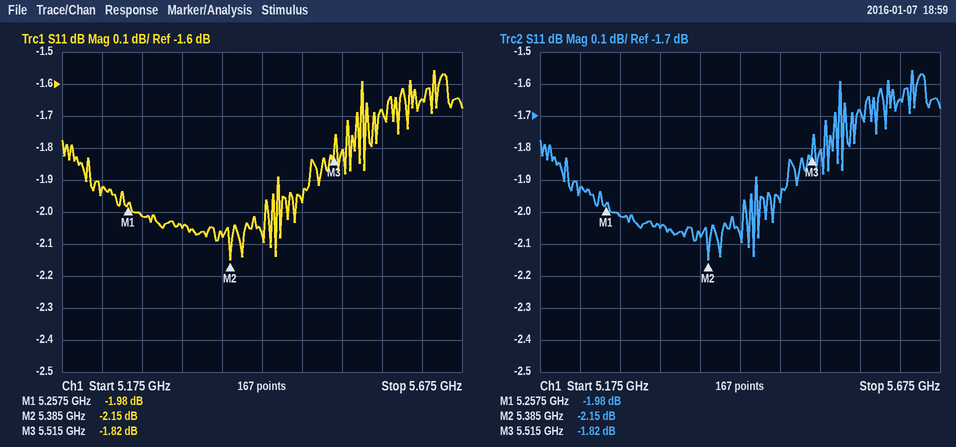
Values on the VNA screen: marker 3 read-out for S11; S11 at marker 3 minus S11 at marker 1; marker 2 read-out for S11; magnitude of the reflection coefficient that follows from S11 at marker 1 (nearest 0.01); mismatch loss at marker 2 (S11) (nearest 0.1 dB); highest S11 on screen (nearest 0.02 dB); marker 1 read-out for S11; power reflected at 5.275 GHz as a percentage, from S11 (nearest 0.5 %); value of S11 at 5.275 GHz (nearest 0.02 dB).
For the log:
-1.82 dB
0.16 dB
-2.15 dB
0.80
4.1 dB
-1.56 dB
-1.98 dB
63.0 %
-2.02 dB
